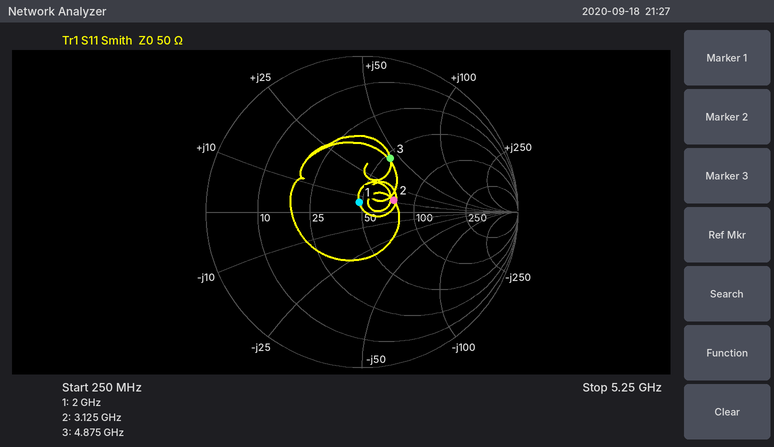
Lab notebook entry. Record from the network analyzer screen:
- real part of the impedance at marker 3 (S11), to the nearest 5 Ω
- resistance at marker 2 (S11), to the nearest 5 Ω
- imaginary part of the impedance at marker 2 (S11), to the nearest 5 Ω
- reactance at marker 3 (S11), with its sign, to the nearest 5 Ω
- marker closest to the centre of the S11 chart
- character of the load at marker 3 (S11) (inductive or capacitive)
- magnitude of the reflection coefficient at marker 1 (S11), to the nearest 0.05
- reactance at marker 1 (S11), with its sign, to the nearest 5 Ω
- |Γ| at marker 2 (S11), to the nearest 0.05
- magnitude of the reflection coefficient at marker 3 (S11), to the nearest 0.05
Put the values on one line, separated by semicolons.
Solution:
55 Ω; 75 Ω; +10 Ω; +45 Ω; marker 1; inductive; 0.05; +5 Ω; 0.20; 0.40
